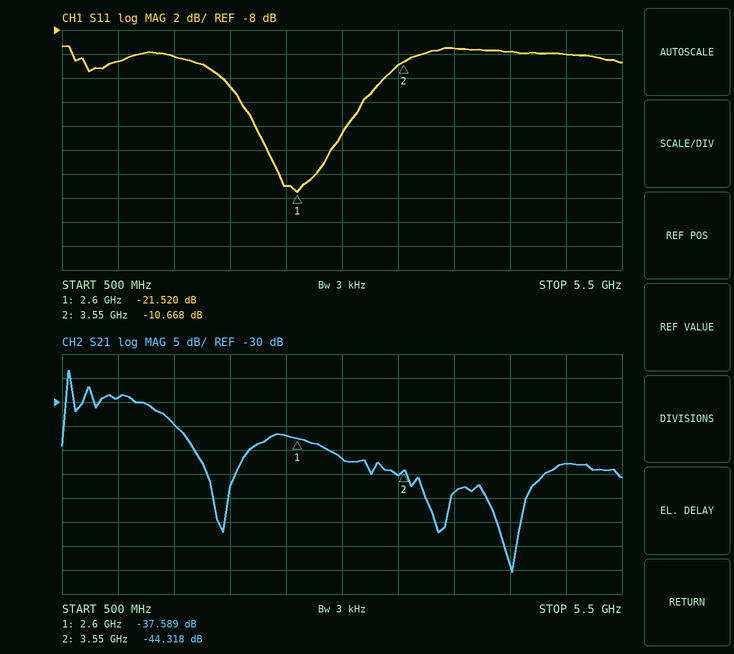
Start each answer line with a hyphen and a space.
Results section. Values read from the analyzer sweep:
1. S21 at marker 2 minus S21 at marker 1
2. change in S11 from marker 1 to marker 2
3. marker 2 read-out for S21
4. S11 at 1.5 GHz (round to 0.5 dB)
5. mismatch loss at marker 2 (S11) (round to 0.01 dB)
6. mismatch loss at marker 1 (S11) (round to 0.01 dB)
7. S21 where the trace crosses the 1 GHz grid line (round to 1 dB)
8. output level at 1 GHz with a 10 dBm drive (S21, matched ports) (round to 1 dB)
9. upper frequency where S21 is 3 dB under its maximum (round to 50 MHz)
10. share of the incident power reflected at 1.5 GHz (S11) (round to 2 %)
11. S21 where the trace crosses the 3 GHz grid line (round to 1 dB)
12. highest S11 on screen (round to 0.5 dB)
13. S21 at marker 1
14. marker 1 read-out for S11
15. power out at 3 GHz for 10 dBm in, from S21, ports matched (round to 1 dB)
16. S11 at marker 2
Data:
- -6.729 dB
- 10.852 dB
- -44.318 dB
- -10.0 dB
- 0.39 dB
- 0.03 dB
- -29 dB
- -19 dBm
- 600 MHz
- 10 %
- -42 dB
- -9.5 dB
- -37.589 dB
- -21.520 dB
- -32 dBm
- -10.668 dB
